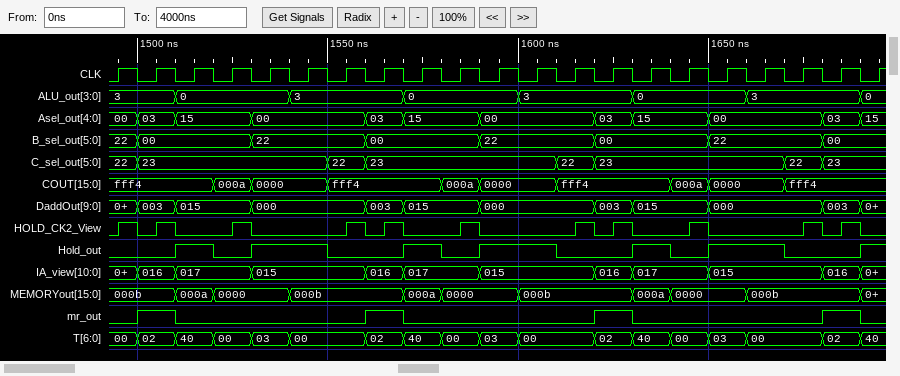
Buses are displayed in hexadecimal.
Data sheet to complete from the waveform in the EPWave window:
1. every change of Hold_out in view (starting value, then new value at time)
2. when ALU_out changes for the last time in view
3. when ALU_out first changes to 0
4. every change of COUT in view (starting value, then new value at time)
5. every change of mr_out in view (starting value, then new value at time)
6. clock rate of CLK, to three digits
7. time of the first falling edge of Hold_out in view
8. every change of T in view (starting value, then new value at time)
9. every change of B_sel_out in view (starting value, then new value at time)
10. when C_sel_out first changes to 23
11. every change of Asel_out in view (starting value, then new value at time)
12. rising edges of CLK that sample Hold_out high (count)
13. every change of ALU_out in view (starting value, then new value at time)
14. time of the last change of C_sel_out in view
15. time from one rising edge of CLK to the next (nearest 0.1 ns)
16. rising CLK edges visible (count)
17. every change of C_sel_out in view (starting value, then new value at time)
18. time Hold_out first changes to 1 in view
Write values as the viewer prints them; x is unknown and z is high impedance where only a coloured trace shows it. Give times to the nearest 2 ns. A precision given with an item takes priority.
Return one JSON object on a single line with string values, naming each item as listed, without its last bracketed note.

{"every change of Hold_out in view": "0, 1 at 1510 ns, 0 at 1520 ns, 1 at 1530 ns, 0 at 1550 ns, 1 at 1570 ns, 0 at 1580 ns, 1 at 1590 ns, 0 at 1610 ns, 1 at 1630 ns, 0 at 1640 ns, 1 at 1650 ns, 0 at 1670 ns, 1 at 1690 ns", "when ALU_out changes for the last time in view": "1690 ns", "when ALU_out first changes to 0": "1510 ns", "every change of COUT in view": "fff4, 000a at 1520 ns, 0000 at 1530 ns, fff4 at 1550 ns, 000a at 1580 ns, 0000 at 1590 ns, fff4 at 1610 ns, 000a at 1640 ns, 0000 at 1650 ns, fff4 at 1670 ns", "every change of mr_out in view": "0, 1 at 1500 ns, 0 at 1510 ns, 1 at 1560 ns, 0 at 1570 ns, 1 at 1620 ns, 0 at 1630 ns, 1 at 1680 ns, 0 at 1690 ns", "clock rate of CLK, to three digits": "100 MHz", "time of the first falling edge of Hold_out in view": "1520 ns", "every change of T in view": "00, 02 at 1500 ns, 40 at 1510 ns, 00 at 1520 ns, 03 at 1530 ns, 00 at 1540 ns, 02 at 1560 ns, 40 at 1570 ns, 00 at 1580 ns, 03 at 1590 ns, 00 at 1600 ns, 02 at 1620 ns, 40 at 1630 ns, 00 at 1640 ns, 03 at 1650 ns, 00 at 1660 ns, 02 at 1680 ns, 40 at 1690 ns", "every change of B_sel_out in view": "22, 00 at 1500 ns, 22 at 1530 ns, 00 at 1560 ns, 22 at 1590 ns, 00 at 1620 ns, 22 at 1650 ns, 00 at 1680 ns", "when C_sel_out first changes to 23": "1500 ns", "every change of Asel_out in view": "00, 03 at 1500 ns, 15 at 1510 ns, 00 at 1530 ns, 03 at 1560 ns, 15 at 1570 ns, 00 at 1590 ns, 03 at 1620 ns, 15 at 1630 ns, 00 at 1650 ns, 03 at 1680 ns, 15 at 1690 ns", "rising edges of CLK that sample Hold_out high": "10", "every change of ALU_out in view": "3, 0 at 1510 ns, 3 at 1540 ns, 0 at 1570 ns, 3 at 1600 ns, 0 at 1630 ns, 3 at 1660 ns, 0 at 1690 ns", "time of the last change of C_sel_out in view": "1680 ns", "time from one rising edge of CLK to the next": "10 ns", "rising CLK edges visible": "21", "every change of C_sel_out in view": "22, 23 at 1500 ns, 22 at 1550 ns, 23 at 1560 ns, 22 at 1610 ns, 23 at 1620 ns, 22 at 1670 ns, 23 at 1680 ns", "time Hold_out first changes to 1 in view": "1510 ns"}
